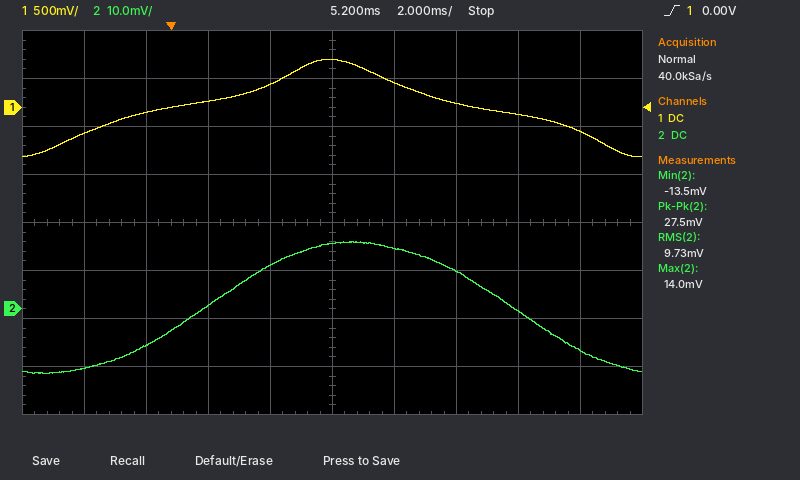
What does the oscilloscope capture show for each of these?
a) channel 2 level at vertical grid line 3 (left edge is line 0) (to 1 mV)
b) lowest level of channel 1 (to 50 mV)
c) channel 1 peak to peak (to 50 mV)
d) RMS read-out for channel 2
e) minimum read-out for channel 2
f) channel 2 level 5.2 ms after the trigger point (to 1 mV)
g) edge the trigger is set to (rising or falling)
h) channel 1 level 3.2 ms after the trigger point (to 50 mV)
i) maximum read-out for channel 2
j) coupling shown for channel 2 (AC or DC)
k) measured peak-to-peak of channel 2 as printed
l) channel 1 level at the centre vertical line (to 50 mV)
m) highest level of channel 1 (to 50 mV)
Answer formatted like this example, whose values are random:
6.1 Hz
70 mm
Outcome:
1 mV
-500 mV
1.00 V
9.73 mV
-13.5 mV
14 mV
rising
250 mV
14.0 mV
DC
27.5 mV
500 mV
500 mV
